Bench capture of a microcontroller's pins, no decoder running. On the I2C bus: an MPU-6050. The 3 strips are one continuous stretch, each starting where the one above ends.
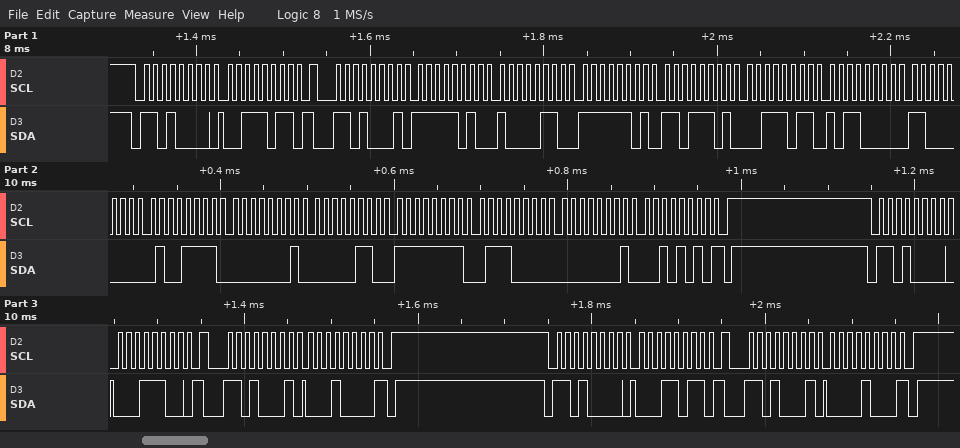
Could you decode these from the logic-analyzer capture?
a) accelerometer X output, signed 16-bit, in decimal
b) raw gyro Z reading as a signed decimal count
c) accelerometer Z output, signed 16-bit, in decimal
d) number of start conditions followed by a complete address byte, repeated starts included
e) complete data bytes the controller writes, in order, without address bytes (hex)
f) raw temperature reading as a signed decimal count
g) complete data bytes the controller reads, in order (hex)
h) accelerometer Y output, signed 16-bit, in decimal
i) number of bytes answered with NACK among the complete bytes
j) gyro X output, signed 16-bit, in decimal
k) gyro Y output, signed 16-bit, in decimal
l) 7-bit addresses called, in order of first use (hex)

-1402
298
15280
6
3B 1C 1B
-16305
FA 86 FD DD 3B B0 C0 4F 01 06 FF 70 01 2A 10 08
-547
3
262
-144
0x68
